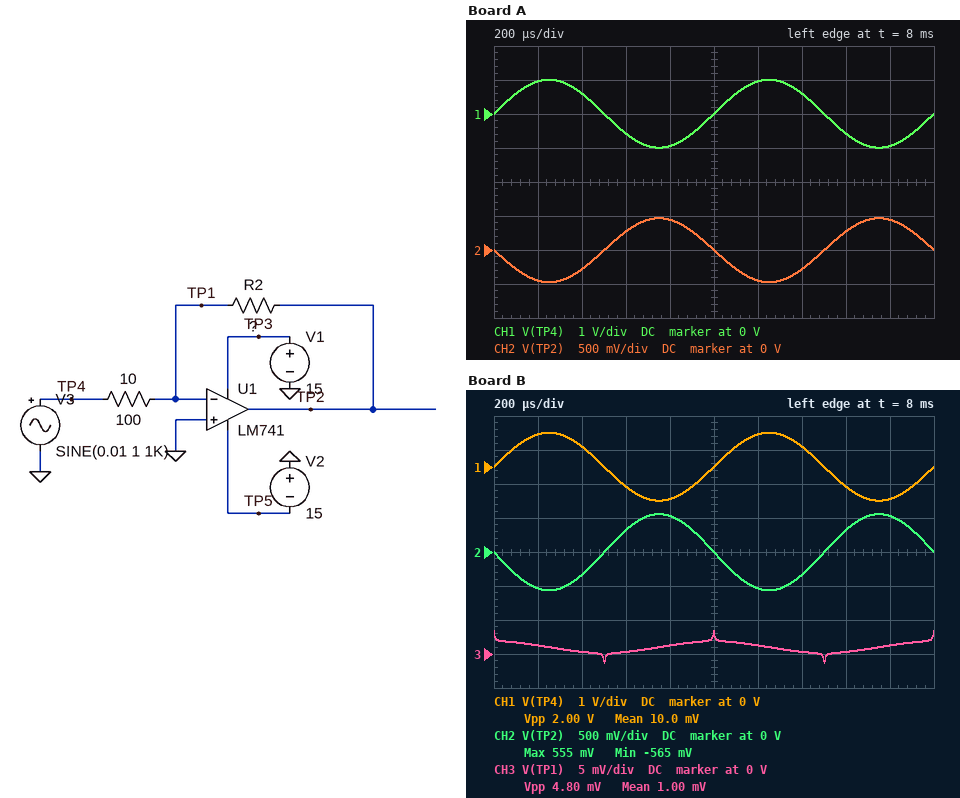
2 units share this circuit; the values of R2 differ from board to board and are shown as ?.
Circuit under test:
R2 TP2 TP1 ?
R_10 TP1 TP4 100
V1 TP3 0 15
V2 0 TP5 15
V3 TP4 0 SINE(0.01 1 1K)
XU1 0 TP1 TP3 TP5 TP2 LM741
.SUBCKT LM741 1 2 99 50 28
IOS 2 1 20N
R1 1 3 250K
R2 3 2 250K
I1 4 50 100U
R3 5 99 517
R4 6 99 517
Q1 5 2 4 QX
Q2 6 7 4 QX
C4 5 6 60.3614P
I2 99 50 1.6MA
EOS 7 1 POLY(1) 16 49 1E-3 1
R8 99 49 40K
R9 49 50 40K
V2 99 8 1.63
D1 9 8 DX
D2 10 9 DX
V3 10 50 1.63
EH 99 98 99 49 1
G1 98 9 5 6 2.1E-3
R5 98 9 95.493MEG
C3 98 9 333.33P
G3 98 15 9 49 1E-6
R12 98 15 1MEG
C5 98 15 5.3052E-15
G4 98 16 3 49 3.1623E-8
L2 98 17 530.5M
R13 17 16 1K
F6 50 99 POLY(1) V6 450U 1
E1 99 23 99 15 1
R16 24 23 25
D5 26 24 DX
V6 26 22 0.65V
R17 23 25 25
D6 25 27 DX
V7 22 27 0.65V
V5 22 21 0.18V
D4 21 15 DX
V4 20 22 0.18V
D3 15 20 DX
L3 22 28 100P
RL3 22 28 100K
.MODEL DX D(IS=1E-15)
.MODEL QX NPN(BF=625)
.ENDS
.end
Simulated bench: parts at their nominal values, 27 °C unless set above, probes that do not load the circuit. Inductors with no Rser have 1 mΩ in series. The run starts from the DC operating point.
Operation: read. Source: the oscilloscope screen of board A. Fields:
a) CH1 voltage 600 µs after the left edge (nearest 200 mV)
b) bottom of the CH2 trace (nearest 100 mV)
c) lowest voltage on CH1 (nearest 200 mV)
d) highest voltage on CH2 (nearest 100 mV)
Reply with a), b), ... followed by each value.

a) -600 mV
b) -500 mV
c) -1.0 V
d) 500 mV
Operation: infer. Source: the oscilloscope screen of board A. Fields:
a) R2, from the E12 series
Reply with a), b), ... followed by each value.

a) 47 Ω
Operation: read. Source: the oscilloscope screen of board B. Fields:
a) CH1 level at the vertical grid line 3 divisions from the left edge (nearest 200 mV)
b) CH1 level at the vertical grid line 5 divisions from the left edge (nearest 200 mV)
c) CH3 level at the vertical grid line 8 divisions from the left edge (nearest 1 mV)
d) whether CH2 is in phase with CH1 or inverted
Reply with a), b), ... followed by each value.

a) -600 mV
b) 0 V
c) 0 V
d) inverted
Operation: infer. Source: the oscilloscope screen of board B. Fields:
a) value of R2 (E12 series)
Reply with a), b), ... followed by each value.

a) 56 Ω
